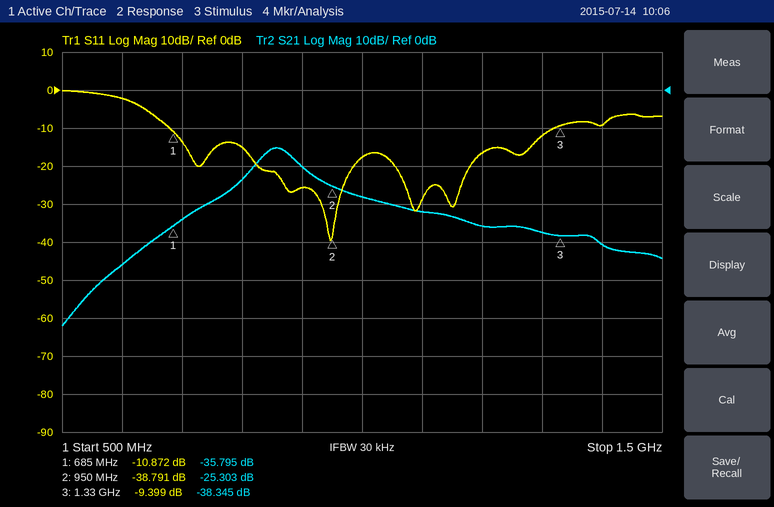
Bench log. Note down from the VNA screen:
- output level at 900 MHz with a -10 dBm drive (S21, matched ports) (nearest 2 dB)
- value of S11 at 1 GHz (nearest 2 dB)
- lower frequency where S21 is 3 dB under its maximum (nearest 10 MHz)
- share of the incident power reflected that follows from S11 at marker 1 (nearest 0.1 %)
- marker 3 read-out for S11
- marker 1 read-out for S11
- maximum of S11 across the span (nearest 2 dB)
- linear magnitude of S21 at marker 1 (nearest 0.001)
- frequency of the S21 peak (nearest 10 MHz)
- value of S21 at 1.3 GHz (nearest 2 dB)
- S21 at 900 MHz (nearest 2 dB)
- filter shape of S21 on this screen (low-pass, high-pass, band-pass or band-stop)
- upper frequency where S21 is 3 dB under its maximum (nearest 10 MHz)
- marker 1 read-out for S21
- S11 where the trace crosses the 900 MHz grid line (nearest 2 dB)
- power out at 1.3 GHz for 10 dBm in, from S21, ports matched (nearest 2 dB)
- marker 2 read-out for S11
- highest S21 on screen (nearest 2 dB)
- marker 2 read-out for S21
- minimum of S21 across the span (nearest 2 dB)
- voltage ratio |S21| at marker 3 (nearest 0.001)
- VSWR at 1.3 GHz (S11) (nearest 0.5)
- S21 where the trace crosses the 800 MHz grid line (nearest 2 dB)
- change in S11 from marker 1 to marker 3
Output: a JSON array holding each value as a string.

["-30 dBm", "-18 dB", "830 MHz", "8.2 %", "-9.399 dB", "-10.872 dB", "0 dB", "0.016", "860 MHz", "-38 dB", "-20 dB", "band-pass", "890 MHz", "-35.795 dB", "-26 dB", "-28 dBm", "-38.791 dB", "-16 dB", "-25.303 dB", "-62 dB", "0.012", "1.5", "-24 dB", "1.473 dB"]
